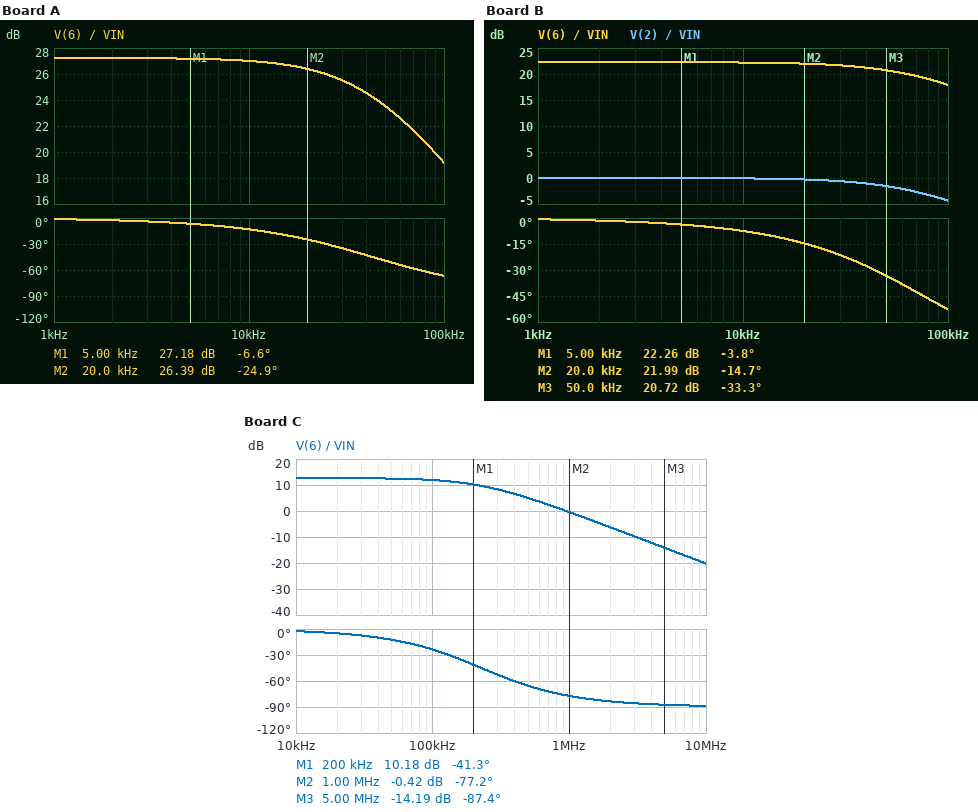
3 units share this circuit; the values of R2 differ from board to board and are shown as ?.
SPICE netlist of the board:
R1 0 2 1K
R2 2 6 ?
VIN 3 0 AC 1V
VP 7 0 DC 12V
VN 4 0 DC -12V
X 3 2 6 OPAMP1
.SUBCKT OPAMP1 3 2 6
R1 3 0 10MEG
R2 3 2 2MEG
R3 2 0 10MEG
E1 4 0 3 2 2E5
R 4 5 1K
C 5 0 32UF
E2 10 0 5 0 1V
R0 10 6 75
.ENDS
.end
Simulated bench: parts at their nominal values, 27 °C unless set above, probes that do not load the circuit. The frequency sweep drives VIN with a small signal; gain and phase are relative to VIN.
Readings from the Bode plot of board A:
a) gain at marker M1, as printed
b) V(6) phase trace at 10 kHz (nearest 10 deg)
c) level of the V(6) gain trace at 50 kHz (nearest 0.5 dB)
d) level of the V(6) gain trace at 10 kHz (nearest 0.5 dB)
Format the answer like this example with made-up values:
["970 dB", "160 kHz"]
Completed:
["27.18 dB", "-10 deg", "23.5 dB", "27.0 dB"]
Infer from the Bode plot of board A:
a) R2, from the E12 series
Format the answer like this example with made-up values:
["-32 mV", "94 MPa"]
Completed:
["22 kΩ"]
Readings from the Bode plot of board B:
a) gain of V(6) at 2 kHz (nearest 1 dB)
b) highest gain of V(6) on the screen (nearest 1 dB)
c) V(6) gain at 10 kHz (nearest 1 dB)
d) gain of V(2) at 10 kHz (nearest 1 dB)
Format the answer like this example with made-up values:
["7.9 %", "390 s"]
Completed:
["22 dB", "22 dB", "22 dB", "0 dB"]
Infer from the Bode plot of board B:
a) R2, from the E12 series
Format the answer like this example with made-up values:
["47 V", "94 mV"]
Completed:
["12 kΩ"]
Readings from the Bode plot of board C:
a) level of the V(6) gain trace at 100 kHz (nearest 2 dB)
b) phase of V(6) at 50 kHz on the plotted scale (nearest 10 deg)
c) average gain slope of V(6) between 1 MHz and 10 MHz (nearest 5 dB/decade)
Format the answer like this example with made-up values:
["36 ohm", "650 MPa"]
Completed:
["12 dB", "-10 deg", "-20 dB/decade"]
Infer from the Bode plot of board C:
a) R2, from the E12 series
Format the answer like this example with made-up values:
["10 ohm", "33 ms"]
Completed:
["3.3 kΩ"]
